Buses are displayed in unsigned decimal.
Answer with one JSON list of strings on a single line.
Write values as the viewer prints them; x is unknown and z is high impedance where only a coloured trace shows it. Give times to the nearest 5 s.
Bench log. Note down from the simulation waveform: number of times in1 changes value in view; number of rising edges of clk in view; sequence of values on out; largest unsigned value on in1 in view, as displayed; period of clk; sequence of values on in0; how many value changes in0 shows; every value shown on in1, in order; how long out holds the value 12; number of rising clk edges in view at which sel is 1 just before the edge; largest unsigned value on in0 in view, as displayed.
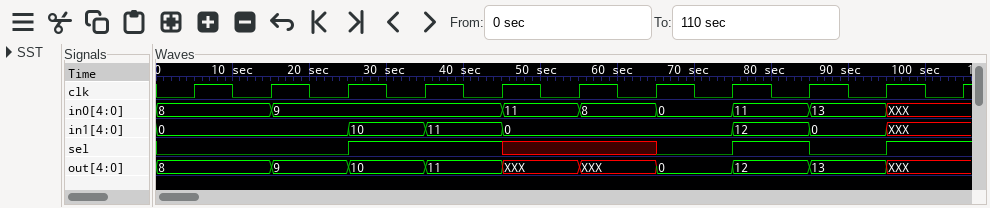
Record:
["6", "11", "8, 9, 10, 11, XXX, XXX, 0, 12, 13, XXX", "12", "10 s", "8, 9, 11, 8, 0, 11, 13, XXX", "7", "0, 10, 11, 0, 12, 0, XXX", "10 s", "4", "13"]
